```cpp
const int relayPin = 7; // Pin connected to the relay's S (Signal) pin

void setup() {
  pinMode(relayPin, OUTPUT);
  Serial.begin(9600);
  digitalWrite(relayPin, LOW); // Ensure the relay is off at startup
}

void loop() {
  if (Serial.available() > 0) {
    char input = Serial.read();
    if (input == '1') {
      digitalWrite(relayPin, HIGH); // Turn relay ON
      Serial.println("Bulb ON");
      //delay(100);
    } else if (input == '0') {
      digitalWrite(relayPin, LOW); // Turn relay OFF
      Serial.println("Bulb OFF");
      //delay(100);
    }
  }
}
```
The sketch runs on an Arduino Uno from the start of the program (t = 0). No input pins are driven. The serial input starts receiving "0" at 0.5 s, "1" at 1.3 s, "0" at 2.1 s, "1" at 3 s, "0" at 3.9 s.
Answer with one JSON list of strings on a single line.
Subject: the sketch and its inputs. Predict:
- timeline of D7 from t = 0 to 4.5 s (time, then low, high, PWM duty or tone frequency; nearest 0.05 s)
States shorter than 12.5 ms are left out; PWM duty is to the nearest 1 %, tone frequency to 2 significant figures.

["0 s low; 1.3 s high; 2.1 s low; 3 s high; 3.9 s low"]
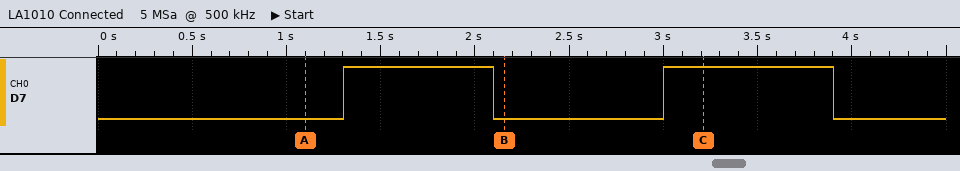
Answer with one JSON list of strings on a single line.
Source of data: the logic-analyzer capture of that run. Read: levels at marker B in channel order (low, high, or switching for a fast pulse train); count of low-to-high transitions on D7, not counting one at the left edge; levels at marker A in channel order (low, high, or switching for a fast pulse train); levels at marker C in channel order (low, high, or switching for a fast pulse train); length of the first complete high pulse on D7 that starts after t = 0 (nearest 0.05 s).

["D7 low", "2", "D7 low", "D7 high", "0.80 s"]
